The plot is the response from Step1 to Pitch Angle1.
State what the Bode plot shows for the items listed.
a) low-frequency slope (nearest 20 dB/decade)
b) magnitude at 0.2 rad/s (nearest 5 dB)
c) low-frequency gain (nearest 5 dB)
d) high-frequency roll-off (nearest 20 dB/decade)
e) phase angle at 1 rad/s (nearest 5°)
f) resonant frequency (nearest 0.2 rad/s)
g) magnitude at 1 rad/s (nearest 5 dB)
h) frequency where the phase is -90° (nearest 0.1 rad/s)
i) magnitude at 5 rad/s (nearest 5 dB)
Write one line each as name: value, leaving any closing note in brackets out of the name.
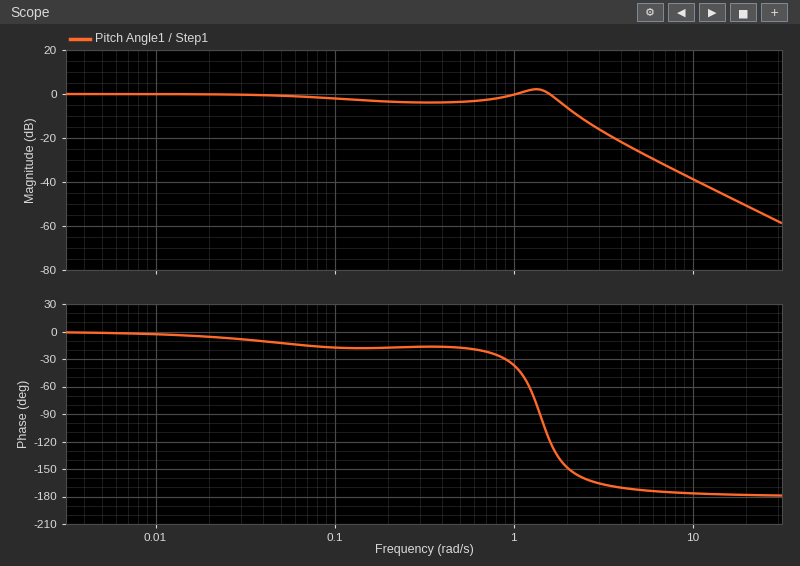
low-frequency slope: 0 dB/decade
magnitude at 0.2 rad/s: -5 dB
low-frequency gain: 0 dB
high-frequency roll-off: -40 dB/decade
phase angle at 1 rad/s: -35°
resonant frequency: 1.4 rad/s
magnitude at 1 rad/s: 0 dB
frequency where the phase is -90°: 1.4 rad/s
magnitude at 5 rad/s: -25 dB
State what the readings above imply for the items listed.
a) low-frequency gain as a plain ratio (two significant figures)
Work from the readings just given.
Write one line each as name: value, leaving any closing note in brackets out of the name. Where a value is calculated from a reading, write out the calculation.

low-frequency gain as a plain ratio: 10^(0 / 20) = 1.0
